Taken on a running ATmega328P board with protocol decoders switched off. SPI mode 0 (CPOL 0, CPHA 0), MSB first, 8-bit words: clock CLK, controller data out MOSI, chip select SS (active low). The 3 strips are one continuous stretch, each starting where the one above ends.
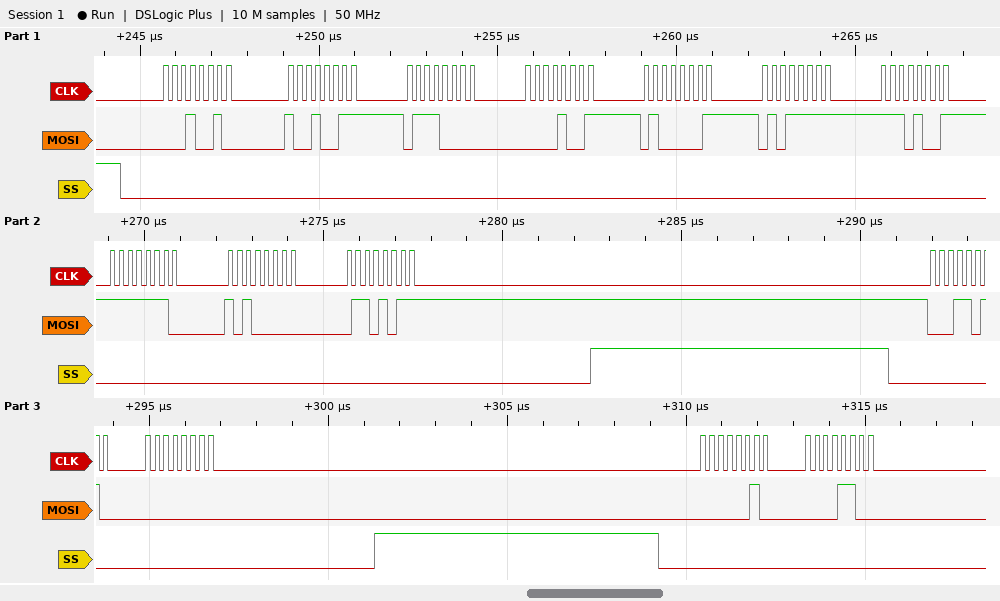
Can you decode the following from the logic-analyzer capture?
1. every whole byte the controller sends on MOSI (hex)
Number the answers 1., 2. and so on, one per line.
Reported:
1. 12 93 70 09 41 5F E9 FE A0 6B 1A 00 02 0C
